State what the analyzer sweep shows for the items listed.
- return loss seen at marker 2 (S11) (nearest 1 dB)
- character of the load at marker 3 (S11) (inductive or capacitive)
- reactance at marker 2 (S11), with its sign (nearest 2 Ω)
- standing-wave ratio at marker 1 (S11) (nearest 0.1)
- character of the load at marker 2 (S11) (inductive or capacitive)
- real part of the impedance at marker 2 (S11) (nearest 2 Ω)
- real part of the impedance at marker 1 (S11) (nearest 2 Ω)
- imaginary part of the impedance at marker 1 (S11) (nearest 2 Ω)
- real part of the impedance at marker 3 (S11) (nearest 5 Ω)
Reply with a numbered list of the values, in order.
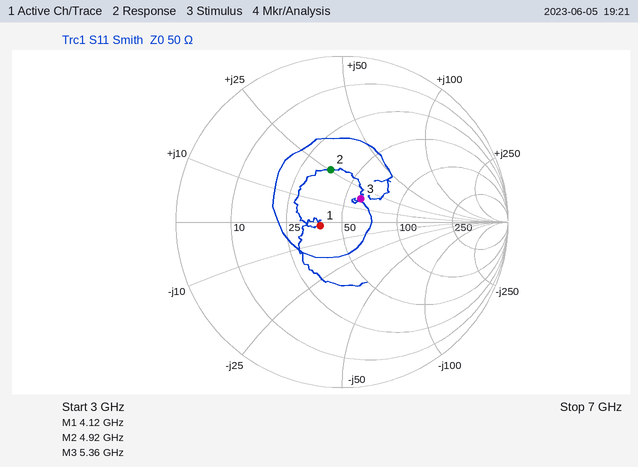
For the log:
1. 10 dB
2. inductive
3. +26 Ω
4. 1.3
5. inductive
6. 36 Ω
7. 38 Ω
8. -2 Ω
9. 60 Ω
